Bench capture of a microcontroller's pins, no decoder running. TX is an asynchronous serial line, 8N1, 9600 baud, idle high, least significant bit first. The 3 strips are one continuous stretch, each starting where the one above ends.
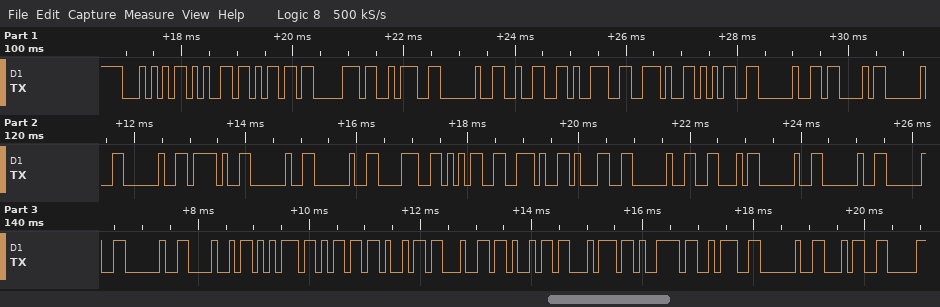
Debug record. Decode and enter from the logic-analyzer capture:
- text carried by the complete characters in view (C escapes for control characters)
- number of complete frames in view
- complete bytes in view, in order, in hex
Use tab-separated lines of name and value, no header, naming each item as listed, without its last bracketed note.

text carried by the complete characters in view	"Temp: 29.5 C  /  85.1 F    Humidity: 4"
number of complete frames in view	38
complete bytes in view, in order, in hex	54 65 6D 70 3A 20 32 39 2E 35 20 43 20 20 2F 20 20 38 35 2E 31 20 46 20 20 20 20 48 75 6D 69 64 69 74 79 3A 20 34
